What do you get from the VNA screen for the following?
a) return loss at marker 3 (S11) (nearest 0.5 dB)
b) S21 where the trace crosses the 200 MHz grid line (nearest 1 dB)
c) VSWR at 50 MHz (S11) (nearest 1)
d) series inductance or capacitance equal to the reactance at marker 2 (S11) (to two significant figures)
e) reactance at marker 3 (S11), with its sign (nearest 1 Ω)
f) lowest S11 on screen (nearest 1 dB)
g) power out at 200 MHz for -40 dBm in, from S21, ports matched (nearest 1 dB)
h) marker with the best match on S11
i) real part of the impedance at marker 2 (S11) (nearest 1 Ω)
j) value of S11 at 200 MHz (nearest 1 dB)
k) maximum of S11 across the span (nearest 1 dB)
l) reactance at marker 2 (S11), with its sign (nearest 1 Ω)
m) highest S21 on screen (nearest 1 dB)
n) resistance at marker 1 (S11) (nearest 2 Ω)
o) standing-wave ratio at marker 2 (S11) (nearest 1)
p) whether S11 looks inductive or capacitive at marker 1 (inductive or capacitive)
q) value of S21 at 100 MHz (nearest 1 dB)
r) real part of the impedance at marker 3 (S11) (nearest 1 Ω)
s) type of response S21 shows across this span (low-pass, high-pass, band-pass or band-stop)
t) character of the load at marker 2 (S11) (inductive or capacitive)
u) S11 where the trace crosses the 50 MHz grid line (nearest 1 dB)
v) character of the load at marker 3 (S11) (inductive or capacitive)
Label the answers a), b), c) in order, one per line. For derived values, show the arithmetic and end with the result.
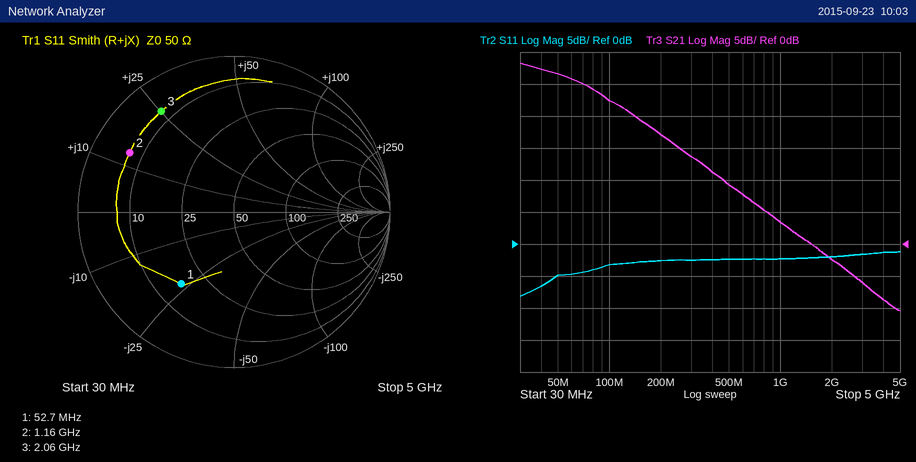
a) 2.0 dB
b) 17 dB
c) |Γ| = 10^(-5/20) = 0.5623; VSWR = (1 + 0.5623)/(1 − 0.5623) ≈ 4
d) L = 13 Ω/(2π × 1.16 GHz) ≈ 1.8 nH
e) +25 Ω
f) -8 dB
g) -40 dBm + (17 dB) = -23 dBm
h) marker 1
i) 7 Ω
j) -3 dB
k) -1 dB
l) +13 Ω
m) 28 dB
n) 16 Ω
o) 8
p) capacitive
q) 22 dB
r) 7 Ω
s) low-pass
t) inductive
u) -5 dB
v) inductive
